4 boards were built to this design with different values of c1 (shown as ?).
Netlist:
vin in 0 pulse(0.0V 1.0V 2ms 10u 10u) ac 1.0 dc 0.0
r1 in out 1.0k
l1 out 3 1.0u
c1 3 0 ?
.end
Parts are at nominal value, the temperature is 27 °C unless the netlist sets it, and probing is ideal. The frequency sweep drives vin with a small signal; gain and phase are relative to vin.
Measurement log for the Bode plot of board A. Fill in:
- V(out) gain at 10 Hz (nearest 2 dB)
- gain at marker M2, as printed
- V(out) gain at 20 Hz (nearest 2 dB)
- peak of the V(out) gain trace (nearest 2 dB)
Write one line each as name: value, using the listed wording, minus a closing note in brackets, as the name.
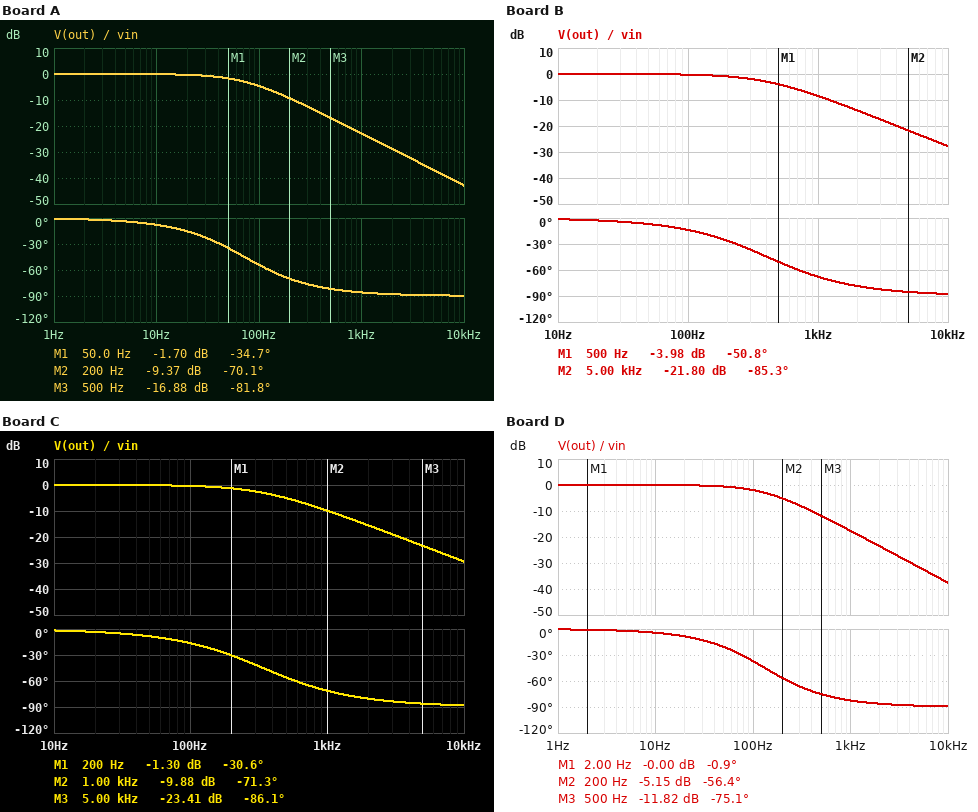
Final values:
V(out) gain at 10 Hz: 0 dB
gain at marker M2, as printed: -9.37 dB
V(out) gain at 20 Hz: 0 dB
peak of the V(out) gain trace: 0 dB
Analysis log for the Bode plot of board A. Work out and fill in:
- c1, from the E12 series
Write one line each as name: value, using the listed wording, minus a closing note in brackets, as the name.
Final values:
c1, from the E12 series: 2.2 µF
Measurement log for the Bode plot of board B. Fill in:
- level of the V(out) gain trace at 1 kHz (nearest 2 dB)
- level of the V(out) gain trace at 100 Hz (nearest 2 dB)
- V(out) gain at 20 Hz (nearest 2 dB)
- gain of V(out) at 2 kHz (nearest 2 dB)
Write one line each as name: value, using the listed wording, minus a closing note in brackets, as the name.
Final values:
level of the V(out) gain trace at 1 kHz: -8 dB
level of the V(out) gain trace at 100 Hz: 0 dB
V(out) gain at 20 Hz: 0 dB
gain of V(out) at 2 kHz: -14 dB
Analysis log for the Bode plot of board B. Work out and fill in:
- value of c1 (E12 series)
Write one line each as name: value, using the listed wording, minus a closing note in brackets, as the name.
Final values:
value of c1: 390 nF
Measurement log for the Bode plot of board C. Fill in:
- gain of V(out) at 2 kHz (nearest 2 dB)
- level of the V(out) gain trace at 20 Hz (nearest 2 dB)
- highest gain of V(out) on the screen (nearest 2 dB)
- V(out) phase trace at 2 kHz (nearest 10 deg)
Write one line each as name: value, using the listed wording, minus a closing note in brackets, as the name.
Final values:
gain of V(out) at 2 kHz: -16 dB
level of the V(out) gain trace at 20 Hz: 0 dB
highest gain of V(out) on the screen: 0 dB
V(out) phase trace at 2 kHz: -80 deg
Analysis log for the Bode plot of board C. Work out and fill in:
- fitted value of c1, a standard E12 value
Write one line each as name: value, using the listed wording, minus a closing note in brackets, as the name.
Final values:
fitted value of c1, a standard E12 value: 470 nF
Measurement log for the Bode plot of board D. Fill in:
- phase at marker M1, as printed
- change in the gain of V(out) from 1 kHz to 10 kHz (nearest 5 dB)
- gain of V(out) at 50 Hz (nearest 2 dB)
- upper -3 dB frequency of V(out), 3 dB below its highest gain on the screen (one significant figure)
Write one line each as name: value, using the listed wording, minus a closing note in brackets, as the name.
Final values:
phase at marker M1, as printed: -0.9 deg
change in the gain of V(out) from 1 kHz to 10 kHz: -20 dB
gain of V(out) at 50 Hz: 0 dB
upper -3 dB frequency of V(out), 3 dB below its highest gain on the screen: 100 Hz
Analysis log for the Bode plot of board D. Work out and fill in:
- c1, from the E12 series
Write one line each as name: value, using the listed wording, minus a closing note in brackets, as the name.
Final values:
c1, from the E12 series: 1.2 µF
